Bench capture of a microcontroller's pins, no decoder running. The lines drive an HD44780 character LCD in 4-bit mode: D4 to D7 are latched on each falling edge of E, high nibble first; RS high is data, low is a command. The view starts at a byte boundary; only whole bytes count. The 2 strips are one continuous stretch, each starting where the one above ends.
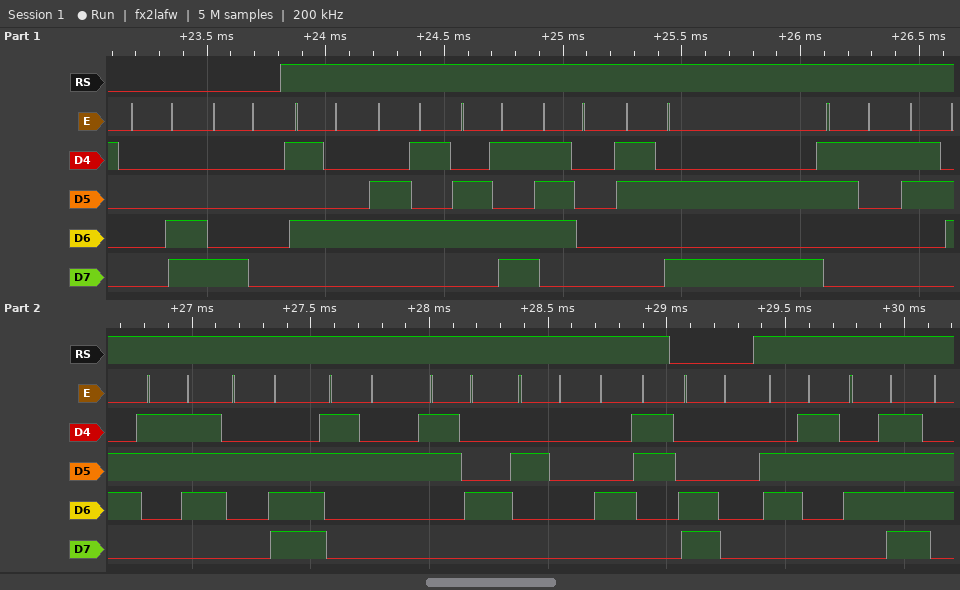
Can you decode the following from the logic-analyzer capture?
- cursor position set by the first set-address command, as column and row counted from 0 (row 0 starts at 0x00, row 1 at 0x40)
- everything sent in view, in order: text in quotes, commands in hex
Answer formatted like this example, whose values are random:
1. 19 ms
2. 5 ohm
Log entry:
1. column 0, row 0
2. 0x0C 0x80 "Temp:167.24 C" 0xC0 "co"
